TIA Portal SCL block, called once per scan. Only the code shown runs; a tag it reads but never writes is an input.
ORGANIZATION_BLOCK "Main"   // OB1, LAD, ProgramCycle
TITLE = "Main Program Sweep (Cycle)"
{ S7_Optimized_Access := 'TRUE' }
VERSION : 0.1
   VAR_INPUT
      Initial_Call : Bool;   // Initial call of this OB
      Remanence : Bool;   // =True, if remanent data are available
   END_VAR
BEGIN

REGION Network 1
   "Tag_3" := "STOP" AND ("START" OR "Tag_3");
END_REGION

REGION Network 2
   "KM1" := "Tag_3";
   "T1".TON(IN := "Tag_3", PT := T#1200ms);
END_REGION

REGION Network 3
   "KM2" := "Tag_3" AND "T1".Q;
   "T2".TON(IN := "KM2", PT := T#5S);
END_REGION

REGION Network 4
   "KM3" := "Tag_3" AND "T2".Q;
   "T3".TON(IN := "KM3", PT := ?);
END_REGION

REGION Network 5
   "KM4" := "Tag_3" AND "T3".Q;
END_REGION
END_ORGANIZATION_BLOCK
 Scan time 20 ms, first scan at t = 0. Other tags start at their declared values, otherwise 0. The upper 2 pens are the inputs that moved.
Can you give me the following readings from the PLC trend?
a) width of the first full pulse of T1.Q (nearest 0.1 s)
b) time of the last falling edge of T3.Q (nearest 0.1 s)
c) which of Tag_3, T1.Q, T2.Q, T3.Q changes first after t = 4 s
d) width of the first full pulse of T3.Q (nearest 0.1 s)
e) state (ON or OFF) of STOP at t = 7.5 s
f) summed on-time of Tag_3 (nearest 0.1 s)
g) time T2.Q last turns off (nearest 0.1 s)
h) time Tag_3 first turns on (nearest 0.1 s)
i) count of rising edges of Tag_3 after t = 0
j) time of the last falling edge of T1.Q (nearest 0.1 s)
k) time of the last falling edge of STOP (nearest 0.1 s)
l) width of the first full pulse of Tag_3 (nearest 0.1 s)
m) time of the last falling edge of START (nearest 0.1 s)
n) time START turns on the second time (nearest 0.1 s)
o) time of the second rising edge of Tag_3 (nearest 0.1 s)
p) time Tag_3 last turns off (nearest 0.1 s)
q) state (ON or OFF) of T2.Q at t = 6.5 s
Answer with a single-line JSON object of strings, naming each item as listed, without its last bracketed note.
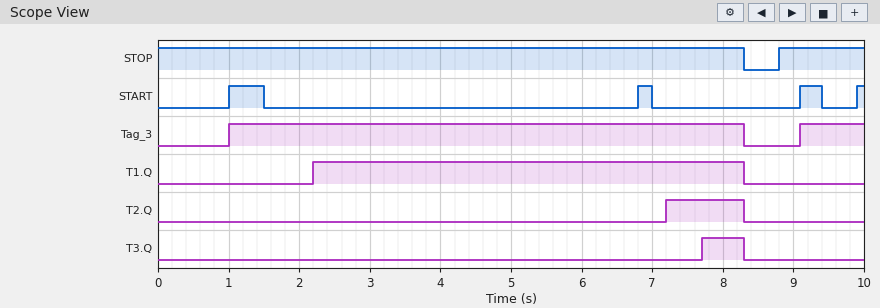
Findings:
{"width of the first full pulse of T1.Q": "6.1 s", "time of the last falling edge of T3.Q": "8.3 s", "which of Tag_3, T1.Q, T2.Q, T3.Q changes first after t = 4 s": "T2.Q", "width of the first full pulse of T3.Q": "0.6 s", "state (ON or OFF) of STOP at t = 7.5 s": "ON", "summed on-time of Tag_3": "8.2 s", "time T2.Q last turns off": "8.3 s", "time Tag_3 first turns on": "1.0 s", "count of rising edges of Tag_3 after t = 0": "2", "time of the last falling edge of T1.Q": "8.3 s", "time of the last falling edge of STOP": "8.3 s", "width of the first full pulse of Tag_3": "7.3 s", "time of the last falling edge of START": "9.4 s", "time START turns on the second time": "6.8 s", "time of the second rising edge of Tag_3": "9.1 s", "time Tag_3 last turns off": "8.3 s", "state (ON or OFF) of T2.Q at t = 6.5 s": "OFF"}
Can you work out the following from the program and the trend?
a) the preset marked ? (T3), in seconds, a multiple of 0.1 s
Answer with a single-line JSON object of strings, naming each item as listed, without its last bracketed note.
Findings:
{"the preset marked ? (T3), in seconds, a multiple of 0.1 s": "0.5 s"}
